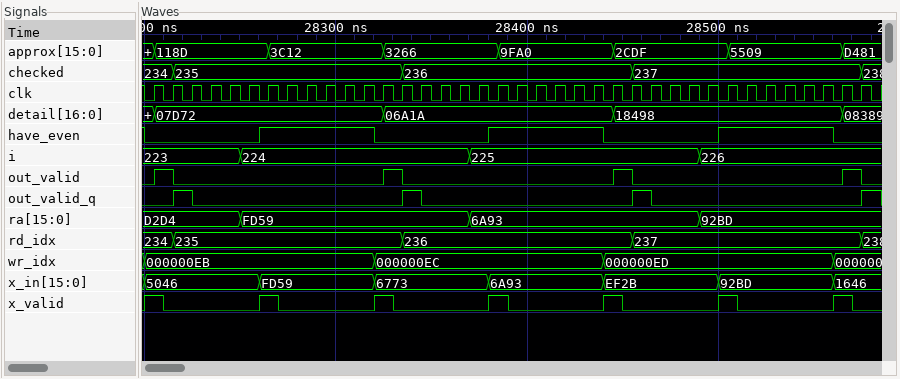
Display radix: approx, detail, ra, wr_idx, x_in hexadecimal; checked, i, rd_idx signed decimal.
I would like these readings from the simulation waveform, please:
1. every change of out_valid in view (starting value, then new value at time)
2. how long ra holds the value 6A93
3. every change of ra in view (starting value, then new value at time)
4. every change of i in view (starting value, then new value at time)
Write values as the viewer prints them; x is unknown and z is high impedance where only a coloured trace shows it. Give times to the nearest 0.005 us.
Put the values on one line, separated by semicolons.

0, 1 at 28.205 us, 0 at 28.215 us, 1 at 28.325 us, 0 at 28.335 us, 1 at 28.445 us, 0 at 28.455 us, 1 at 28.565 us, 0 at 28.575 us; 0.12 us; D2D4, FD59 at 28.25 us, 6A93 at 28.37 us, 92BD at 28.49 us; 223, 224 at 28.25 us, 225 at 28.37 us, 226 at 28.49 us
